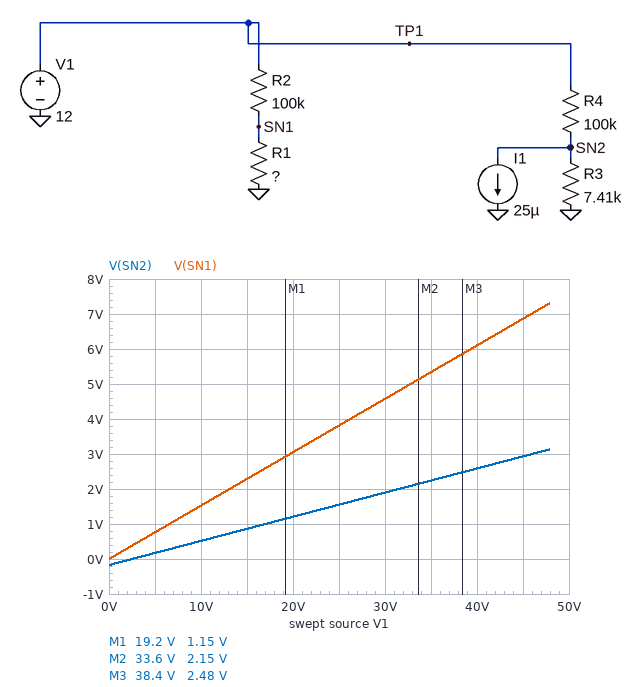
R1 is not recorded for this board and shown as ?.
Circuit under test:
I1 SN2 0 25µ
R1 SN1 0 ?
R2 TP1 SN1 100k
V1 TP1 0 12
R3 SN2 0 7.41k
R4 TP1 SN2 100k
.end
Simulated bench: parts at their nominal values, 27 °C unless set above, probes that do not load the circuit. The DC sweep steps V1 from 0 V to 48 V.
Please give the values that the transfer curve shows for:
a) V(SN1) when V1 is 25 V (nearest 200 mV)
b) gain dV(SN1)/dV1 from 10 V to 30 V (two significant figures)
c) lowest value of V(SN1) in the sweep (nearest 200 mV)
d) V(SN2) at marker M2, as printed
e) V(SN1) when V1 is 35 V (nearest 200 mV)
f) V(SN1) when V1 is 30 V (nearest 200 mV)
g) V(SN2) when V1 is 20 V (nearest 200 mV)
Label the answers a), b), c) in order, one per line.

a) 3.8 V
b) 0.15 V/V
c) 0 V
d) 2.15 V
e) 5.4 V
f) 4.6 V
g) 1.2 V
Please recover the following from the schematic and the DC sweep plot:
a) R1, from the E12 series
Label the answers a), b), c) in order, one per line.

a) 18 kΩ
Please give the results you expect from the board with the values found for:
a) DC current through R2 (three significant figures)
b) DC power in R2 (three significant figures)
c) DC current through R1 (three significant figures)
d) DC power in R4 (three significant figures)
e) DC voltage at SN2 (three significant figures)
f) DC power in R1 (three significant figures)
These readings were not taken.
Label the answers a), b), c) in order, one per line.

a) 102 µA
b) 1.03 mW
c) 102 µA
d) 1.29 mW
e) 655 mV
f) 186 µW
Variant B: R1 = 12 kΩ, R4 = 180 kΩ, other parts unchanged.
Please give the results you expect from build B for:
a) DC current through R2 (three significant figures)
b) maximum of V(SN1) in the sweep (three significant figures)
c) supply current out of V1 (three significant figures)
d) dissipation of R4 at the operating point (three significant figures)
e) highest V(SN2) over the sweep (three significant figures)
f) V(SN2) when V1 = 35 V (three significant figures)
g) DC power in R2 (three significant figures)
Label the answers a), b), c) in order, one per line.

a) 107 µA
b) 5.14 V
c) 172 µA
d) 761 µW
e) 1.72 V
f) 1.21 V
g) 1.15 mW
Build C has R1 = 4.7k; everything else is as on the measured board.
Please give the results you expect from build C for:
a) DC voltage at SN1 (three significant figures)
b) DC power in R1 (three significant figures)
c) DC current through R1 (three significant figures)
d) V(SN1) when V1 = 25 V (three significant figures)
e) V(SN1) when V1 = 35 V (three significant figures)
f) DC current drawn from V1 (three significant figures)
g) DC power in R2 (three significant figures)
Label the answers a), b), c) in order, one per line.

a) 539 mV
b) 61.7 µW
c) 115 µA
d) 1.12 V
e) 1.57 V
f) 228 µA
g) 1.31 mW
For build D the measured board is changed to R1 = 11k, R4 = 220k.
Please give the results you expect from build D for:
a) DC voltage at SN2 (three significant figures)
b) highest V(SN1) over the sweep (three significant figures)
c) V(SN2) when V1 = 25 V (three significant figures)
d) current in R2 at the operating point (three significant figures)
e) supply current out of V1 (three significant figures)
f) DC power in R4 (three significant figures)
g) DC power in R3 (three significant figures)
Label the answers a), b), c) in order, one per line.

a) 212 mV
b) 4.76 V
c) 635 mV
d) 108 µA
e) 162 µA
f) 632 µW
g) 6.05 µW
